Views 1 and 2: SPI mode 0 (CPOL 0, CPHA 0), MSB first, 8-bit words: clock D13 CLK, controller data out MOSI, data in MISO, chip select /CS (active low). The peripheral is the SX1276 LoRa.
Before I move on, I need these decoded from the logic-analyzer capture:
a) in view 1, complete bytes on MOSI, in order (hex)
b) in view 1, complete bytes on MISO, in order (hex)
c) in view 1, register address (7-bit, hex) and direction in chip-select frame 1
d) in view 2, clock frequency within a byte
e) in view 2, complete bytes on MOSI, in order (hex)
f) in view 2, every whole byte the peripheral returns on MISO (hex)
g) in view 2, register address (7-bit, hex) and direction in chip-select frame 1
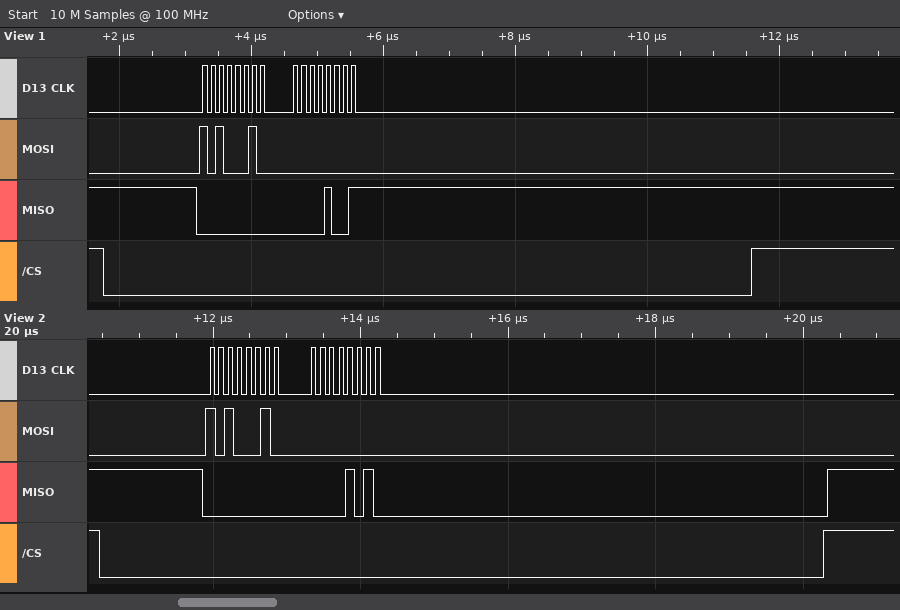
A2 00
00 09
0x22 write
8 MHz
0xA2 0x00
0x00 0x0A
0x22 write
